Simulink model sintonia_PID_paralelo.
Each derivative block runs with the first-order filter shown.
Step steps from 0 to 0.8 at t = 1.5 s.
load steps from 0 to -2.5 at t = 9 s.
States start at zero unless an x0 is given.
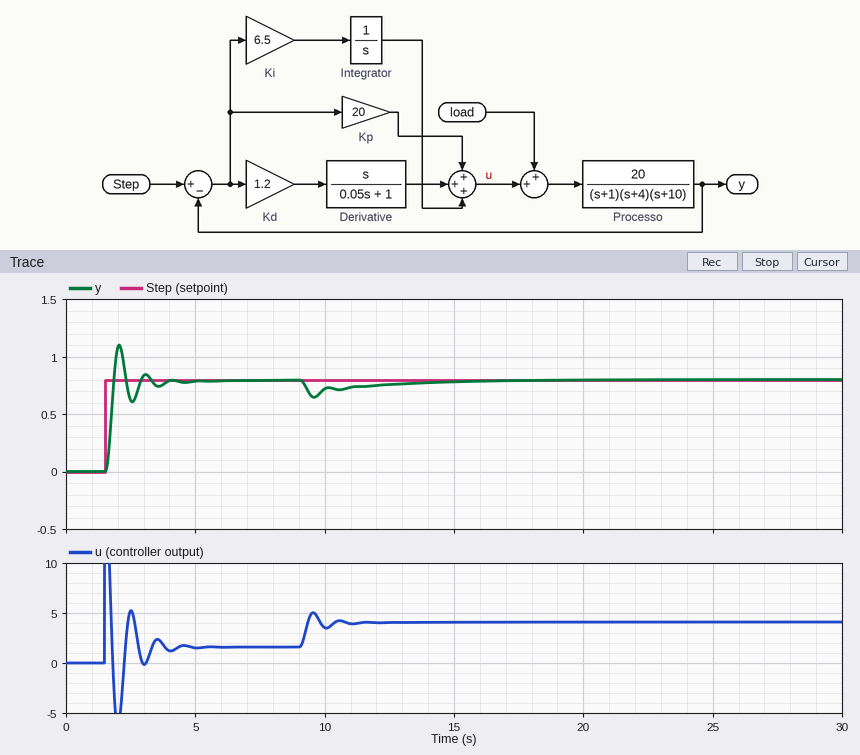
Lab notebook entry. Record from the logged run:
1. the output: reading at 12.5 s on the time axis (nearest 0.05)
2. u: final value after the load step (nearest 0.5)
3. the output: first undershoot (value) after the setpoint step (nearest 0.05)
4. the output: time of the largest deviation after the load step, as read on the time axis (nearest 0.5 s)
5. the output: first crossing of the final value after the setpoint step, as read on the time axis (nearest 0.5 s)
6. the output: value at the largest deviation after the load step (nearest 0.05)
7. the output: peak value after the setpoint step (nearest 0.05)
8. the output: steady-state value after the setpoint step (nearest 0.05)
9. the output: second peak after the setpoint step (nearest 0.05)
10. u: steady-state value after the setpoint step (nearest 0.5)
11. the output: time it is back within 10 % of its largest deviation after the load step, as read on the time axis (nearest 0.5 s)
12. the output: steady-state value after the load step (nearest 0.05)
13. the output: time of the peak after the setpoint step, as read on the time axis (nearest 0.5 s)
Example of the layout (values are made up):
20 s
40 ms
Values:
0.75
4.0
0.60
9.5 s
2.0 s
0.65
1.10
0.80
0.85
1.5
16.0 s
0.80
2.0 s
